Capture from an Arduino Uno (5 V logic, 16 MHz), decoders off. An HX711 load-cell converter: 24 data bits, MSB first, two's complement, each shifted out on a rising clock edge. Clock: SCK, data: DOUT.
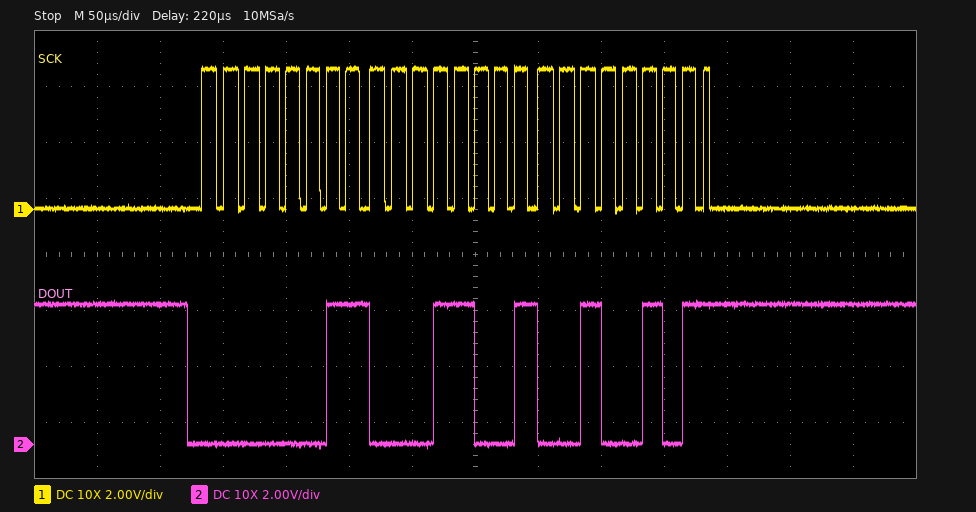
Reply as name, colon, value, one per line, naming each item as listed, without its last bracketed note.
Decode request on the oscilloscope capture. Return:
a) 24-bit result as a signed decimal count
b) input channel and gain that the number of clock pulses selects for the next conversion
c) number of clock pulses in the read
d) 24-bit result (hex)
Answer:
24-bit result as a signed decimal count: 203045
input channel and gain that the number of clock pulses selects for the next conversion: channel A, gain 128
number of clock pulses in the read: 25
24-bit result: 0x031925
